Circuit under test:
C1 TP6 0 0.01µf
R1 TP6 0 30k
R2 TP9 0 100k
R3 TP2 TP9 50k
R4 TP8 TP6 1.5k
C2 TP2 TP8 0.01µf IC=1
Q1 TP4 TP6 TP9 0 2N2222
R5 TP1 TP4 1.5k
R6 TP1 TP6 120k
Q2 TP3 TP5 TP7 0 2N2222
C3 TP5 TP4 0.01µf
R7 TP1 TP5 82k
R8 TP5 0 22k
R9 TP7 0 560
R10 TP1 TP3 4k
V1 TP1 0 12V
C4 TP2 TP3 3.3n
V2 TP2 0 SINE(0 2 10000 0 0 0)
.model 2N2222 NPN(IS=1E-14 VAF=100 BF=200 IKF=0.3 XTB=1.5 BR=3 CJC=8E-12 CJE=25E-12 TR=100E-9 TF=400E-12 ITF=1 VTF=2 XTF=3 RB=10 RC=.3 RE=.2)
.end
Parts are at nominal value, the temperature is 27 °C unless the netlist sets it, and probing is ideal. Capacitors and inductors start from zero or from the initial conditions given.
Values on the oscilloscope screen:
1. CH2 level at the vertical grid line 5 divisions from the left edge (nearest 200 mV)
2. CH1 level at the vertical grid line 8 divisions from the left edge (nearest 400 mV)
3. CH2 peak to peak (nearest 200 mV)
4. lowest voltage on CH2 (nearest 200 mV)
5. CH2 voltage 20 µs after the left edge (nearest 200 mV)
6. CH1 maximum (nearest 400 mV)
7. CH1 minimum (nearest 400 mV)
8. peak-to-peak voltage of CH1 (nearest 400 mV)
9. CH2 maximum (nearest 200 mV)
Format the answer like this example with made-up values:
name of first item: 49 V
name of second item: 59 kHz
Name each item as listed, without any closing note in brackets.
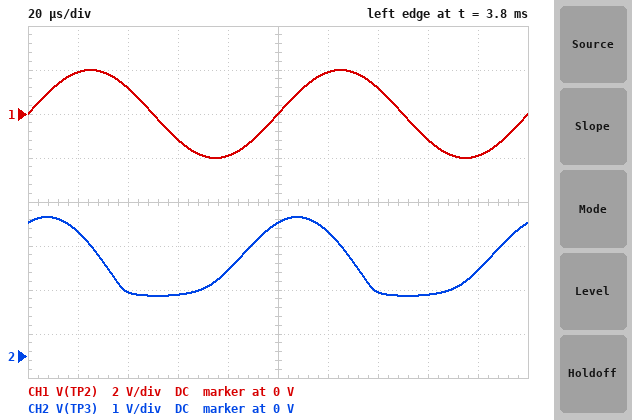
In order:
CH2 level at the vertical grid line 5 divisions from the left edge: 3.0 V
CH1 level at the vertical grid line 8 divisions from the left edge: -1.2 V
CH2 peak to peak: 1.8 V
lowest voltage on CH2: 1.4 V
CH2 voltage 20 µs after the left edge: 2.8 V
CH1 maximum: 2.0 V
CH1 minimum: -2.0 V
peak-to-peak voltage of CH1: 4.0 V
CH2 maximum: 3.2 V
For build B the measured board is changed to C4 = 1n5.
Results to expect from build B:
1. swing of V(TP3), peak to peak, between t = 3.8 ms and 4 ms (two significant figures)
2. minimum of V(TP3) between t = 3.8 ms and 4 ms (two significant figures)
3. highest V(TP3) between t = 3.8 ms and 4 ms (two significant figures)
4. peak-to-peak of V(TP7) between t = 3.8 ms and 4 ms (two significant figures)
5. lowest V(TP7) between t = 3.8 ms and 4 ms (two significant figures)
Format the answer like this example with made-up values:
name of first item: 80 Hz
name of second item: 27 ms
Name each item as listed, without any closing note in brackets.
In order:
swing of V(TP3), peak to peak, between t = 3.8 ms and 4 ms: 710 mV
minimum of V(TP3) between t = 3.8 ms and 4 ms: 1.5 V
highest V(TP3) between t = 3.8 ms and 4 ms: 2.2 V
peak-to-peak of V(TP7) between t = 3.8 ms and 4 ms: 120 mV
lowest V(TP7) between t = 3.8 ms and 4 ms: 1.4 V
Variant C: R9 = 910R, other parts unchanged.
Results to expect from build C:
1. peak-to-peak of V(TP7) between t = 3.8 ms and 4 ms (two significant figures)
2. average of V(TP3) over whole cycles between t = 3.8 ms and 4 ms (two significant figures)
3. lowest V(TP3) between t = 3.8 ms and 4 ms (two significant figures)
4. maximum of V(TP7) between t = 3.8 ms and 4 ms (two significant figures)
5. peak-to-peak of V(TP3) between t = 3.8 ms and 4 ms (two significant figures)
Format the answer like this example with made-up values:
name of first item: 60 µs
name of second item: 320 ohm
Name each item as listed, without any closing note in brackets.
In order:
peak-to-peak of V(TP7) between t = 3.8 ms and 4 ms: 51 mV
average of V(TP3) over whole cycles between t = 3.8 ms and 4 ms: 4.5 V
lowest V(TP3) between t = 3.8 ms and 4 ms: 3.3 V
maximum of V(TP7) between t = 3.8 ms and 4 ms: 1.7 V
peak-to-peak of V(TP3) between t = 3.8 ms and 4 ms: 2.4 V
